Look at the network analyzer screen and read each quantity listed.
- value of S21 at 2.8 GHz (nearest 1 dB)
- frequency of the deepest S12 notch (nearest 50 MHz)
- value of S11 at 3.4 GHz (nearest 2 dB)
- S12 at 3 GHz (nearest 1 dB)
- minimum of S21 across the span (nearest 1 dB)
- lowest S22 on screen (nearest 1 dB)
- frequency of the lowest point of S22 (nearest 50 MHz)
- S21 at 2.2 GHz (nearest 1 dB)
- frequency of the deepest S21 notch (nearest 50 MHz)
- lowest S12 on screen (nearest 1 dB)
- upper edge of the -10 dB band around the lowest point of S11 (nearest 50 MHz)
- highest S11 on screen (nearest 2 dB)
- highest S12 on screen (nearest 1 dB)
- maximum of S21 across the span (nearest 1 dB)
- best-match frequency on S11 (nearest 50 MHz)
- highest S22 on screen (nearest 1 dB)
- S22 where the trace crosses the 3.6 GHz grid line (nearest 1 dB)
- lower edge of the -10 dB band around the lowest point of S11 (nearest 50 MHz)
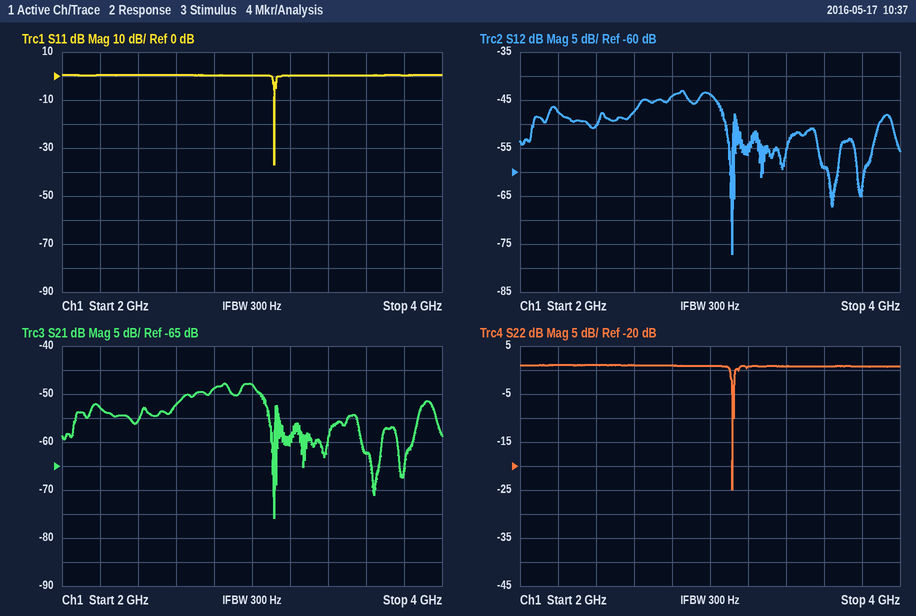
-49 dB
3.10 GHz
0 dB
-44 dB
-76 dB
-25 dB
3.10 GHz
-53 dB
3.10 GHz
-77 dB
3.10 GHz
0 dB
-43 dB
-48 dB
3.10 GHz
1 dB
1 dB
3.10 GHz
